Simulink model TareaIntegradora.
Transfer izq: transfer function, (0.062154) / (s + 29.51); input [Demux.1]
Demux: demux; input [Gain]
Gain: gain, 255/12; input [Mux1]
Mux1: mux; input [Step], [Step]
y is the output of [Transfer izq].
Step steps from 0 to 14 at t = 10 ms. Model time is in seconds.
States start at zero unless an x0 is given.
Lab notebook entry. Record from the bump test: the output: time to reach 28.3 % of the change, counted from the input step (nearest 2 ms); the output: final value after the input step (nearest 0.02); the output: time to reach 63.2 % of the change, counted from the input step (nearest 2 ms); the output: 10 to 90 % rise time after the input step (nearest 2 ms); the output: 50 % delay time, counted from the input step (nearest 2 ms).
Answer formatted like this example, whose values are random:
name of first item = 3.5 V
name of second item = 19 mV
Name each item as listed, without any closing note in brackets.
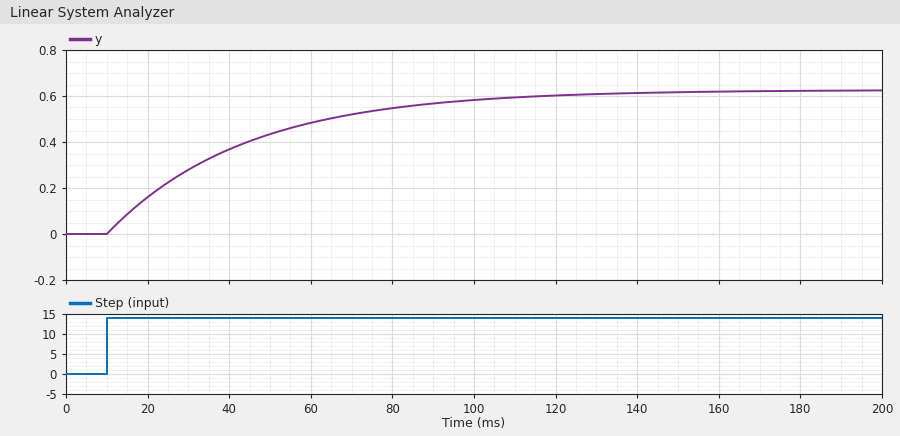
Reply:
the output: time to reach 28.3 % of the change, counted from the input step = 12 ms
the output: final value after the input step = 0.62
the output: time to reach 63.2 % of the change, counted from the input step = 34 ms
the output: 10 to 90 % rise time after the input step = 74 ms
the output: 50 % delay time, counted from the input step = 24 ms
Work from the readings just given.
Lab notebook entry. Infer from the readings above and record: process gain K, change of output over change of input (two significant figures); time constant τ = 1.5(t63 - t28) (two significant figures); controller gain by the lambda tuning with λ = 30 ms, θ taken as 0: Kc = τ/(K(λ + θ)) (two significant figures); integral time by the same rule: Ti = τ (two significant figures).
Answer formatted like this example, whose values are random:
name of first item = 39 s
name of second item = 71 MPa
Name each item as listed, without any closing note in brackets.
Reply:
process gain K, change of output over change of input = 0.044
time constant τ = 1.5(t63 - t28) = 33 ms
controller gain by the lambda tuning with λ = 30 ms, θ taken as 0: Kc = τ/(K(λ + θ)) = 25
integral time by the same rule: Ti = τ = 33 ms
